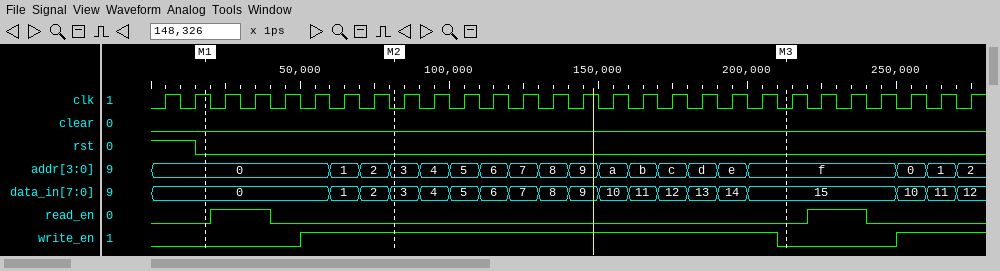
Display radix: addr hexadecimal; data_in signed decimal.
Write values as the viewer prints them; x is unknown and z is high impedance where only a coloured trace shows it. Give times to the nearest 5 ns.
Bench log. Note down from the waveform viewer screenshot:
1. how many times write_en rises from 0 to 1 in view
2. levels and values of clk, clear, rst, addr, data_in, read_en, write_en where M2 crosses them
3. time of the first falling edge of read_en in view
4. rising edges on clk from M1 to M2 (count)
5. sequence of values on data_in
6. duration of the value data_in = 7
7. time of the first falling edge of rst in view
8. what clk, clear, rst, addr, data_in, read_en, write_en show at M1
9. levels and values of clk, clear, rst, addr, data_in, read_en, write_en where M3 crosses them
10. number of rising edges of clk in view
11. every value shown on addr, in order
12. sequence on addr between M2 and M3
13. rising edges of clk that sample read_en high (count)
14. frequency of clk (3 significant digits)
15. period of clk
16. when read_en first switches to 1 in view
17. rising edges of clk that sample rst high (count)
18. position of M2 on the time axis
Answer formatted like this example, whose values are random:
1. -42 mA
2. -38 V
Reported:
1. 2
2. clk=0, clear=0, rst=0, addr=3, data_in=3, read_en=0, write_en=1
3. 40 ns
4. 6
5. 0, 1, 2, 3, 4, 5, 6, 7, 8, 9, 10, 11, 12, 13, 14, 15, 10, 11, 12
6. 10 ns
7. 15 ns
8. clk=1, clear=0, rst=0, addr=0, data_in=0, read_en=0, write_en=0
9. clk=0, clear=0, rst=0, addr=f, data_in=15, read_en=0, write_en=0
10. 28
11. 0, 1, 2, 3, 4, 5, 6, 7, 8, 9, a, b, c, d, e, f, 0, 1, 2
12. 3, 4, 5, 6, 7, 8, 9, a, b, c, d, e, f
13. 4
14. 100 MHz
15. 10 ns
16. 20 ns
17. 2
18. 80 ns
